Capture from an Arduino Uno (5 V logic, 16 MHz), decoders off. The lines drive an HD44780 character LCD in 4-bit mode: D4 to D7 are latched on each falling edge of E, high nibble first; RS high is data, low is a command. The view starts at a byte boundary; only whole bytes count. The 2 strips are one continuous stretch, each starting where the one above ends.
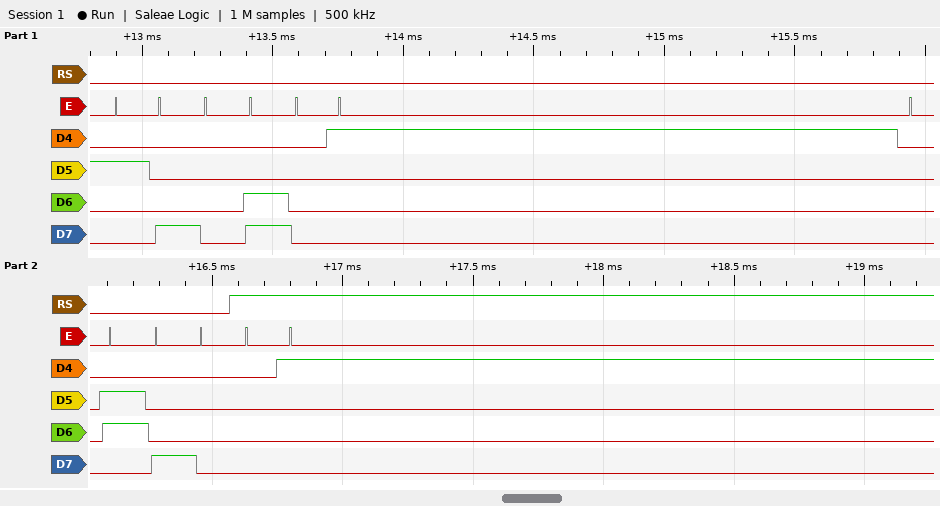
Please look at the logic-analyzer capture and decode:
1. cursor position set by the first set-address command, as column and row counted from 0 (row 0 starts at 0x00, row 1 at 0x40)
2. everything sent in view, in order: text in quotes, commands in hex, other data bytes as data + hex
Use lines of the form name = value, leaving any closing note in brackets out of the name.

cursor position set by the first set-address command, as column and row counted from 0 = column 0, row 0
everything sent in view, in order: text in quotes, commands in hex, other data bytes as data + hex = 0x28 0x0C 0x01 0x06 0x80 data 01
